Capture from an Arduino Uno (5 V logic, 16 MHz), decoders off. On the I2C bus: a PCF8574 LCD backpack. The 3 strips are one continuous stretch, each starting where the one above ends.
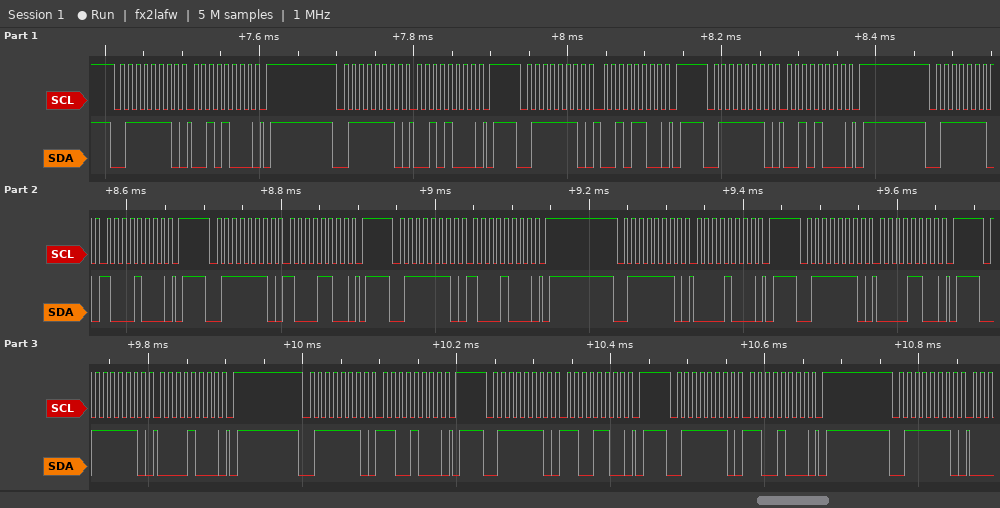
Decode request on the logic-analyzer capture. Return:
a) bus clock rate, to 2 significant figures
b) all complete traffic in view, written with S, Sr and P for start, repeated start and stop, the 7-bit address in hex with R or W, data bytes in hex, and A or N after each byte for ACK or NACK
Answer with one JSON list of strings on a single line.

["100 kHz", "S 3FW A 28 A P S 3FW A 28 A P S 3FW A 2C A P S 3FW A 28 A P S 3FW A 88 A P S 3FW A 8C A P S 3FW A 88 A P S 3FW A 08 A P S 3FW A 0C A P S 3FW A 08 A P S 3FW A C8 A P S 3FW A CC A P S 3FW A C8 A P S 3FW A"]
